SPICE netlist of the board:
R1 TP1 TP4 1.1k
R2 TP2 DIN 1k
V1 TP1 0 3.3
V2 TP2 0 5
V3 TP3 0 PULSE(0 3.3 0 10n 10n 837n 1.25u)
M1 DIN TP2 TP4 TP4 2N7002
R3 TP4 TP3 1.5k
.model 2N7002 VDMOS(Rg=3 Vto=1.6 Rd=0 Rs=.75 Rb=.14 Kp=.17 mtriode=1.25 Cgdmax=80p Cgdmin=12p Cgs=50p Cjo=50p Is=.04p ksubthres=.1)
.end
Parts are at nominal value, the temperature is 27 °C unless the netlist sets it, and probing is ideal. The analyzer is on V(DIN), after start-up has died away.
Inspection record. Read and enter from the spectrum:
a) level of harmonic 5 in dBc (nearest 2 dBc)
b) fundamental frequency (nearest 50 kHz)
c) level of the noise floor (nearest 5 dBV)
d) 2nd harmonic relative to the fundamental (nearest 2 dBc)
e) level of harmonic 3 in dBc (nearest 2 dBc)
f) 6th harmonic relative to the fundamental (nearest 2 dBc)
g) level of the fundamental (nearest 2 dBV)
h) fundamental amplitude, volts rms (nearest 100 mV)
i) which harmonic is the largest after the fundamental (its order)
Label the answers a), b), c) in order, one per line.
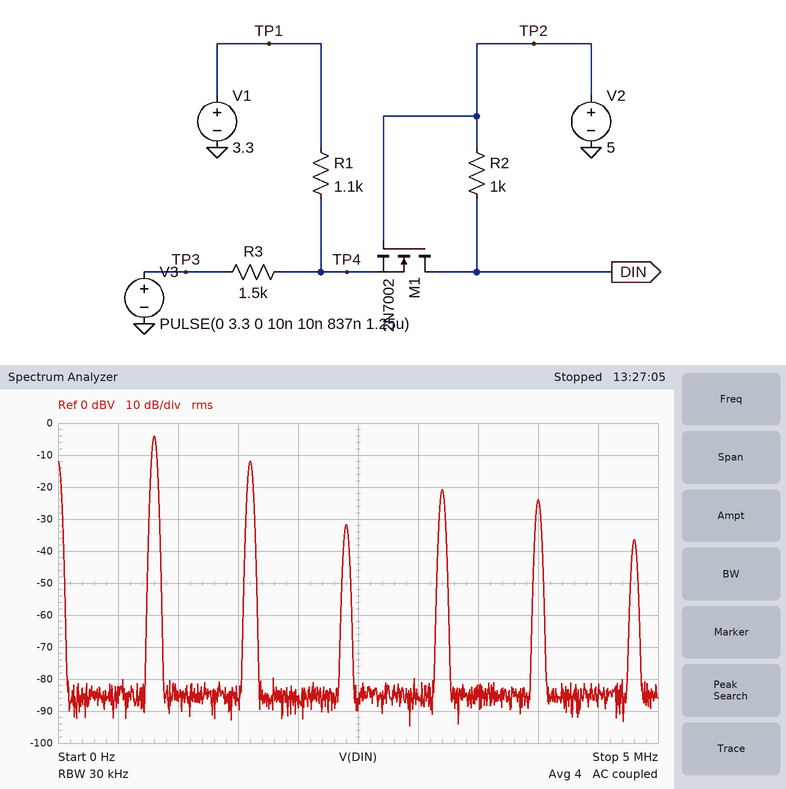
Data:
a) -20 dBc
b) 800 kHz
c) -85 dBV
d) -8 dBc
e) -28 dBc
f) -32 dBc
g) -4 dBV
h) 600 mV
i) 2
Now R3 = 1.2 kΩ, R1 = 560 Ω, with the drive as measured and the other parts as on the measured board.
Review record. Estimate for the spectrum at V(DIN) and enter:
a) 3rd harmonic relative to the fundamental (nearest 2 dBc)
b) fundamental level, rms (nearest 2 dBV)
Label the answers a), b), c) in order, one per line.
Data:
a) -24 dBc
b) -4 dBV
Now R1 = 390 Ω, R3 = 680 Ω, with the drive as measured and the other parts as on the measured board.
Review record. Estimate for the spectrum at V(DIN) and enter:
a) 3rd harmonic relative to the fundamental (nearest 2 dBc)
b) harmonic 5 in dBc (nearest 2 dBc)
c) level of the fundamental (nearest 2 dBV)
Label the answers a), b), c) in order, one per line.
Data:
a) -22 dBc
b) -18 dBc
c) -2 dBV
